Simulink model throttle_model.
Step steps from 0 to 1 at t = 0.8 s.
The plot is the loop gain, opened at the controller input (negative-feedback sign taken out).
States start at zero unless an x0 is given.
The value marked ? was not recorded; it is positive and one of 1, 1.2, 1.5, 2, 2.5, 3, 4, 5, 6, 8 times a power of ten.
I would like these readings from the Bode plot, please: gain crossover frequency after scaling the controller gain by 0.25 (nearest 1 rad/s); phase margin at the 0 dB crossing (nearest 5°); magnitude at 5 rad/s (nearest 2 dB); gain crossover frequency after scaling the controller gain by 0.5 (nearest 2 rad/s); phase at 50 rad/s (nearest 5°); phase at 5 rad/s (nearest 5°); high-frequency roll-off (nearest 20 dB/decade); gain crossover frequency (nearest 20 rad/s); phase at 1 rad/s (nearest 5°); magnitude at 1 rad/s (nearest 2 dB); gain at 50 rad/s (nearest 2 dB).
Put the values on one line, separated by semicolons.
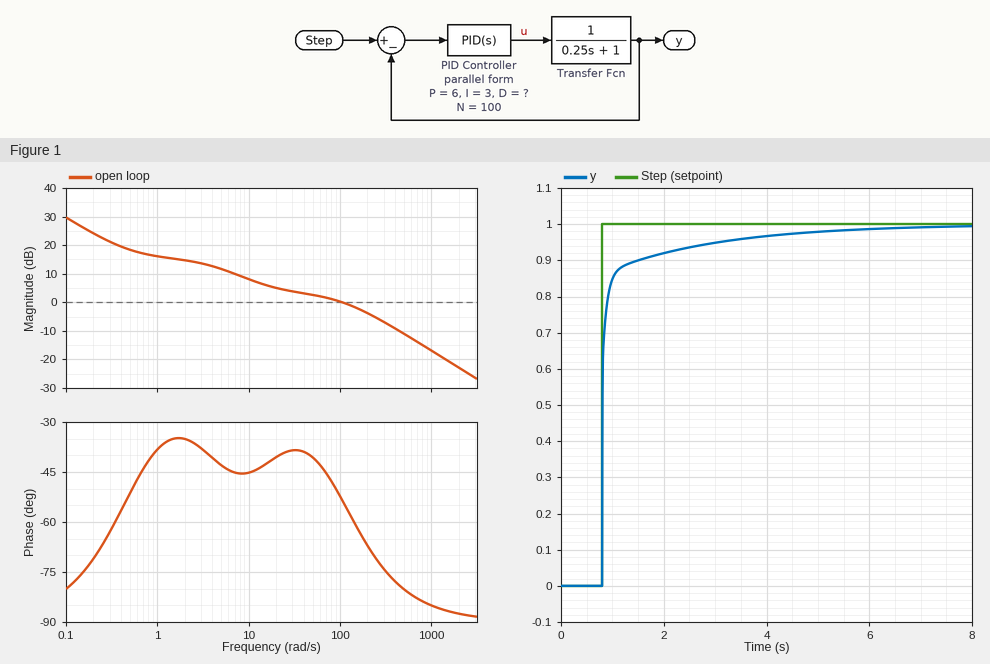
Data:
5 rad/s; 125°; 12 dB; 16 rad/s; -40°; -45°; -20 dB/decade; 100 rad/s; -40°; 16 dB; 2 dB
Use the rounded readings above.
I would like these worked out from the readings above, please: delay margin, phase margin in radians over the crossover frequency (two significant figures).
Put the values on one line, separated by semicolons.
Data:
0.022 s
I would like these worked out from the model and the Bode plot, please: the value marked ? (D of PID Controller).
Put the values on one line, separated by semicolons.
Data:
0.3
